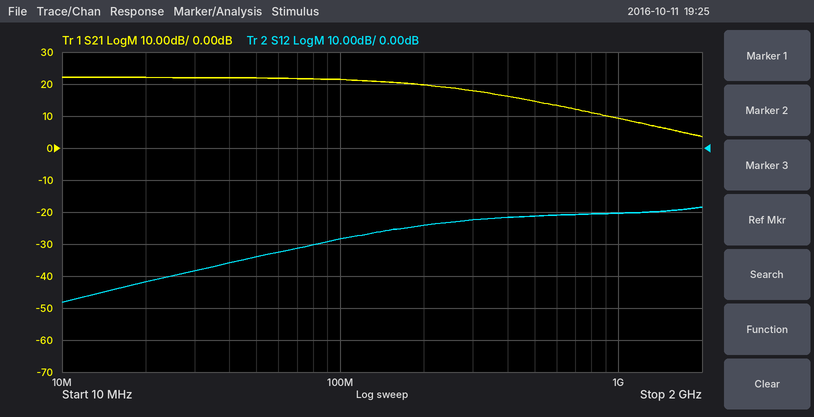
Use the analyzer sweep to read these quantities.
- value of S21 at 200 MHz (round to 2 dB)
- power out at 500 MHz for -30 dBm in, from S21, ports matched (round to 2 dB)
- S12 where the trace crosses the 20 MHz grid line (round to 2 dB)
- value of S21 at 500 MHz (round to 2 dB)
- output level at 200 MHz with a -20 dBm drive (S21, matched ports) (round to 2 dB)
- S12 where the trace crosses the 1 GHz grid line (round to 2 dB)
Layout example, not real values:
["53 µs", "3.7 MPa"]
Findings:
["20 dB", "-16 dBm", "-42 dB", "14 dB", "0 dBm", "-20 dB"]
